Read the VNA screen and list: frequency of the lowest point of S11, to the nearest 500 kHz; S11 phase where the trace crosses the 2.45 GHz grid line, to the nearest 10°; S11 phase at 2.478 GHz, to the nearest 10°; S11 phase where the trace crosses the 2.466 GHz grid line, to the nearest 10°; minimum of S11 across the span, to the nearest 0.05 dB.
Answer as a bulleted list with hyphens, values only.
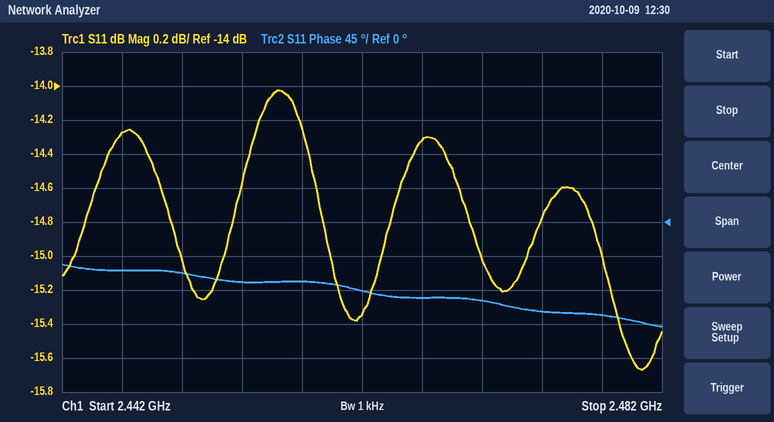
- 2.4805 GHz
- -70°
- -120°
- -100°
- -15.65 dB
